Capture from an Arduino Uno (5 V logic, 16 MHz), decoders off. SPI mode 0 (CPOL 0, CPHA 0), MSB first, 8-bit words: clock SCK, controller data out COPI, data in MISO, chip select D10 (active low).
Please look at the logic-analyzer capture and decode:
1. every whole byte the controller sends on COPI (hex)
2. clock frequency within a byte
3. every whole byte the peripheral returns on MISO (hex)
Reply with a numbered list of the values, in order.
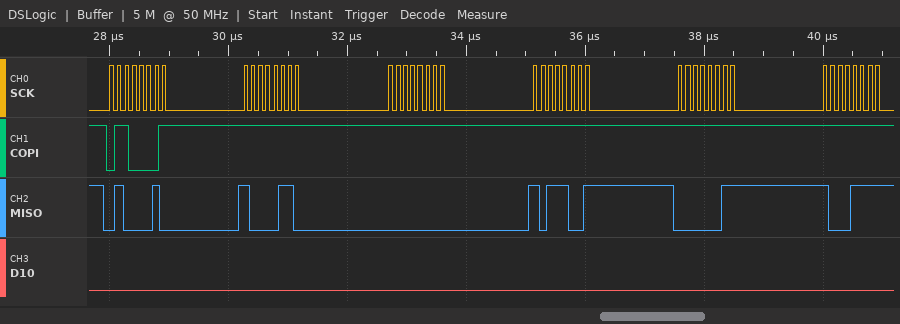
1. 0x61 0xFF 0xFF 0xFF 0xFF 0xFF
2. 8 MHz
3. 0x42 0x86 0x00 0xB9 0x03 0x8F
